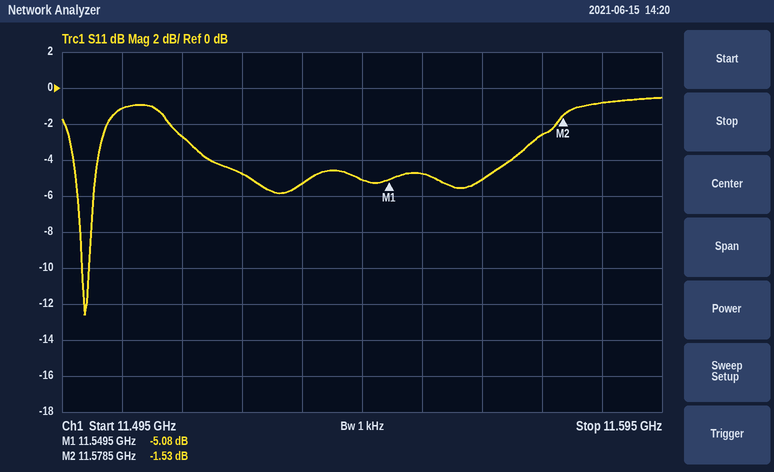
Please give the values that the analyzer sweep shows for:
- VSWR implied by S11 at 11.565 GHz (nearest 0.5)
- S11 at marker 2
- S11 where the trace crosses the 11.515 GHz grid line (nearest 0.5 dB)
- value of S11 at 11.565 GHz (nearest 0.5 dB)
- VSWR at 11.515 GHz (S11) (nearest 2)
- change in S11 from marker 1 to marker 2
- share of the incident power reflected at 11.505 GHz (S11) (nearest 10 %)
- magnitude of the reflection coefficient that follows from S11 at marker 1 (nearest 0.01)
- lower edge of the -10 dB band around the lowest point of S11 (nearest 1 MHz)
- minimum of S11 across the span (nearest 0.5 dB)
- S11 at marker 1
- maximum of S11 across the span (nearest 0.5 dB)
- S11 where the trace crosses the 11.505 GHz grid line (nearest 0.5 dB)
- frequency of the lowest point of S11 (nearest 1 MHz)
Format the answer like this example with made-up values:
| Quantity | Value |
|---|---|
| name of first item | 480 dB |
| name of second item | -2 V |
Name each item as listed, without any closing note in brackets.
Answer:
| Quantity | Value |
|---|---|
| VSWR implied by S11 at 11.565 GHz | 3.5 |
| S11 at marker 2 | -1.53 dB |
| S11 where the trace crosses the 11.515 GHz grid line | -2.5 dB |
| value of S11 at 11.565 GHz | -5.0 dB |
| VSWR at 11.515 GHz (S11) | 6 |
| change in S11 from marker 1 to marker 2 | 3.55 dB |
| share of the incident power reflected at 11.505 GHz (S11) | 80 % |
| magnitude of the reflection coefficient that follows from S11 at marker 1 | 0.56 |
| lower edge of the -10 dB band around the lowest point of S11 | 11.498 GHz |
| minimum of S11 across the span | -12.5 dB |
| S11 at marker 1 | -5.08 dB |
| maximum of S11 across the span | -0.5 dB |
| S11 where the trace crosses the 11.505 GHz grid line | -1.0 dB |
| frequency of the lowest point of S11 | 11.499 GHz |
